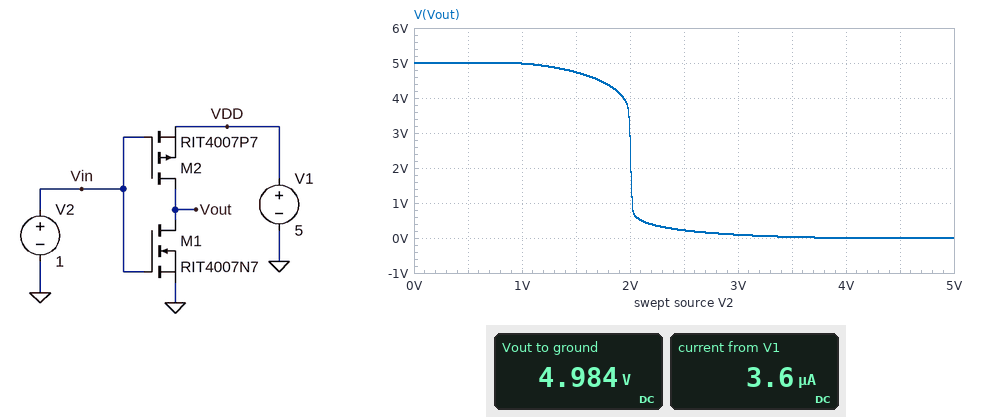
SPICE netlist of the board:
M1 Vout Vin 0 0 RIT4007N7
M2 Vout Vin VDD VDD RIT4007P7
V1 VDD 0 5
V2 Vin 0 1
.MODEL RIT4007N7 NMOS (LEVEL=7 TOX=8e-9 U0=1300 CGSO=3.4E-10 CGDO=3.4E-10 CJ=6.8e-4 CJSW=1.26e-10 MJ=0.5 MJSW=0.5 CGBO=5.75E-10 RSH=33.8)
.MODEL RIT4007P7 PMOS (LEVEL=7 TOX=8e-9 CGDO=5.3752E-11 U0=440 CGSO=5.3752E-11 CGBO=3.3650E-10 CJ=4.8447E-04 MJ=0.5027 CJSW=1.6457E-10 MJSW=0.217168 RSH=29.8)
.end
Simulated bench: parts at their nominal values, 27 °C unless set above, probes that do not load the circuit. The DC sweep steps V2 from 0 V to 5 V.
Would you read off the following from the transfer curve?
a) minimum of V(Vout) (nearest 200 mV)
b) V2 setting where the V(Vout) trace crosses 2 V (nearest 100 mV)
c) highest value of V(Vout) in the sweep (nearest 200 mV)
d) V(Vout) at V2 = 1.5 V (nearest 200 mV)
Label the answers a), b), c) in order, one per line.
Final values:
a) 0 V
b) 2.0 V
c) 5.0 V
d) 4.8 V
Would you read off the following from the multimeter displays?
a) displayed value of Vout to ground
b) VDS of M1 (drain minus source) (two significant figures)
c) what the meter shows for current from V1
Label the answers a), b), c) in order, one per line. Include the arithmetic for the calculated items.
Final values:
a) 4.984 V
b) 4.984 V = 5.0 V
c) 3.6 µA
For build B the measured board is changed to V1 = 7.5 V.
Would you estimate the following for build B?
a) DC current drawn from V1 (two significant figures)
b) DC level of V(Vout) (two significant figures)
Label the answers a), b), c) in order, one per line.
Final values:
a) 5.5 µA
b) 7.5 V
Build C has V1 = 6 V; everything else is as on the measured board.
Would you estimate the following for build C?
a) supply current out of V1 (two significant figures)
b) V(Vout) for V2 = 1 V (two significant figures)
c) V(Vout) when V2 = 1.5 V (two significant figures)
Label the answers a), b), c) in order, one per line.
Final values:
a) 4.1 µA
b) 6.0 V
c) 5.8 V
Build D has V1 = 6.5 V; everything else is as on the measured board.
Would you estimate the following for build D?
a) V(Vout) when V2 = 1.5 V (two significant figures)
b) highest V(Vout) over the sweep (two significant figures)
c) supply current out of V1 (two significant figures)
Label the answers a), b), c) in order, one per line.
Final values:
a) 6.3 V
b) 6.5 V
c) 4.5 µA
